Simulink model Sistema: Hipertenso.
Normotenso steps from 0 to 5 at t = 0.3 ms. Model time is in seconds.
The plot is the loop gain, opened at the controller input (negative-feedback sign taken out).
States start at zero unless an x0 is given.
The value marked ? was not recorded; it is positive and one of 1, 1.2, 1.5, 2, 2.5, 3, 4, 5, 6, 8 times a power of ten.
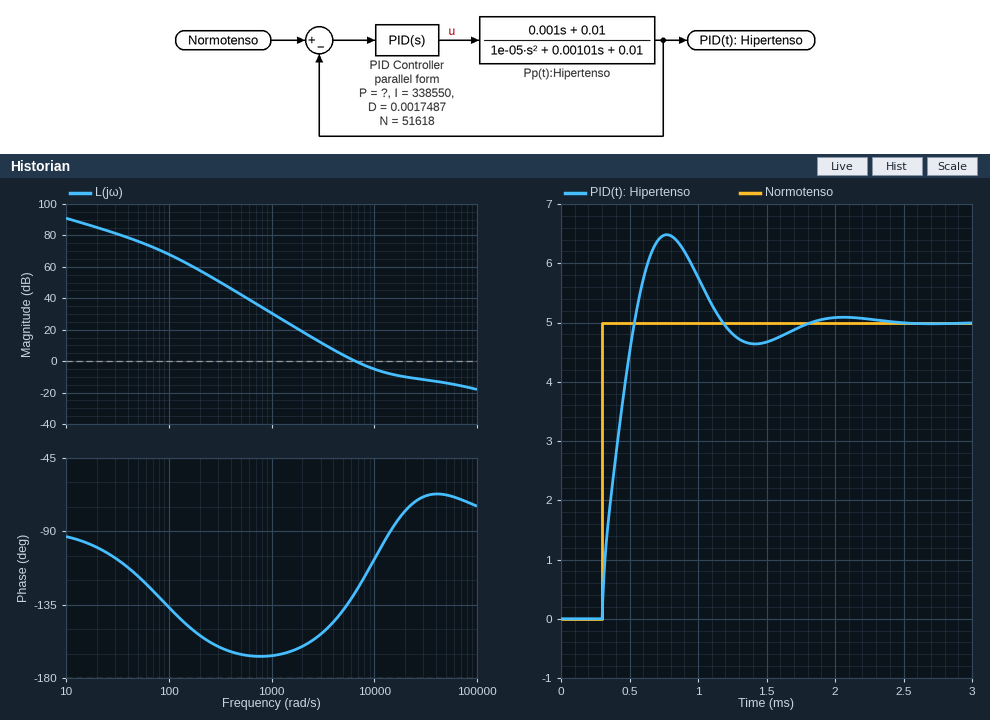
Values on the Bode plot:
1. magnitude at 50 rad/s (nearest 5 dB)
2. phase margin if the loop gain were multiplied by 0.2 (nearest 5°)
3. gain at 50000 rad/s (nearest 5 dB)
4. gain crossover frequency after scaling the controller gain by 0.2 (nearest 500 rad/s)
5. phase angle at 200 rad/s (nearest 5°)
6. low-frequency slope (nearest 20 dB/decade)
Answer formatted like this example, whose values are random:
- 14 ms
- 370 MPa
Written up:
- 75 dB
- 25°
- -15 dB
- 2500 rad/s
- -155°
- -20 dB/decade
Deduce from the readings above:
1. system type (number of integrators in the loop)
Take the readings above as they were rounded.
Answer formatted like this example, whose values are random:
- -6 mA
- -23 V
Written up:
- 1
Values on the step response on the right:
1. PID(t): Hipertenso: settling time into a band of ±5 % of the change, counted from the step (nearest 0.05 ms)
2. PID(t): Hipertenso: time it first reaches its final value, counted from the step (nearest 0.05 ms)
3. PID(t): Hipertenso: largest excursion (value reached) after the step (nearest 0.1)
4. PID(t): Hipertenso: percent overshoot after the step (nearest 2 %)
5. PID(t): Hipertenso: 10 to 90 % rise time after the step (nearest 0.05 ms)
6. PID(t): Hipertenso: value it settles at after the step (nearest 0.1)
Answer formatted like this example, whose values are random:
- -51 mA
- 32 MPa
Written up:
- 1.30 ms
- 0.25 ms
- 6.5
- 30 %
- 0.20 ms
- 5.0
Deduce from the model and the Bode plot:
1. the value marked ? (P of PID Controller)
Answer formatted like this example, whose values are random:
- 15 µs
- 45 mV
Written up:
- 50
